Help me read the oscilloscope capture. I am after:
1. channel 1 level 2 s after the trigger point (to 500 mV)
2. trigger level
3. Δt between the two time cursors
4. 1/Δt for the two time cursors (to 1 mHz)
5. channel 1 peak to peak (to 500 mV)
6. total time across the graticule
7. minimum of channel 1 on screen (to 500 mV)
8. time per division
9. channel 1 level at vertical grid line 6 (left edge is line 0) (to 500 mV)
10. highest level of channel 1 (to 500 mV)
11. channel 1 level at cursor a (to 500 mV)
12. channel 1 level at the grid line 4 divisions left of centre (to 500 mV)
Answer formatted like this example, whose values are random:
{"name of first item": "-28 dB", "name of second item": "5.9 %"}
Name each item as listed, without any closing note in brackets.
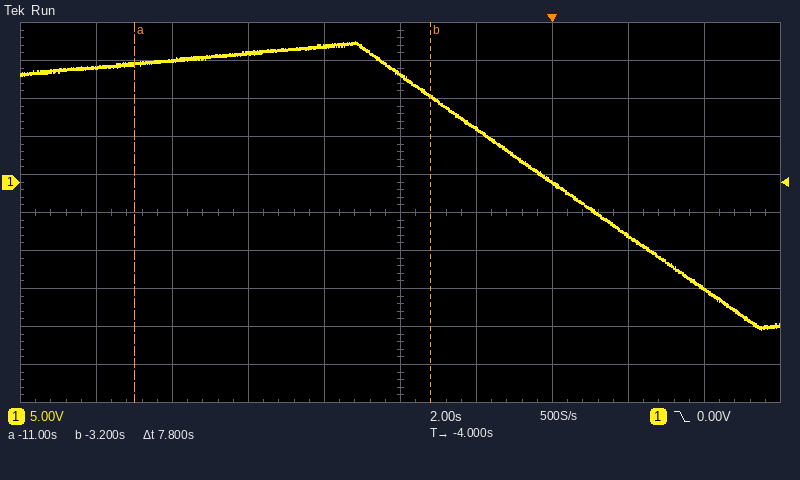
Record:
{"channel 1 level 2 s after the trigger point": "-7.0 V", "trigger level": "0.00 V", "Δt between the two time cursors": "7.8 s", "1/Δt for the two time cursors": "128 mHz", "channel 1 peak to peak": "38.0 V", "total time across the graticule": "20 s", "minimum of channel 1 on screen": "-19.5 V", "time per division": "2 s", "channel 1 level at vertical grid line 6 (left edge is line 0)": "7.0 V", "highest level of channel 1": "18.5 V", "channel 1 level at cursor a": "15.5 V", "channel 1 level at the grid line 4 divisions left of centre": "15.0 V"}
